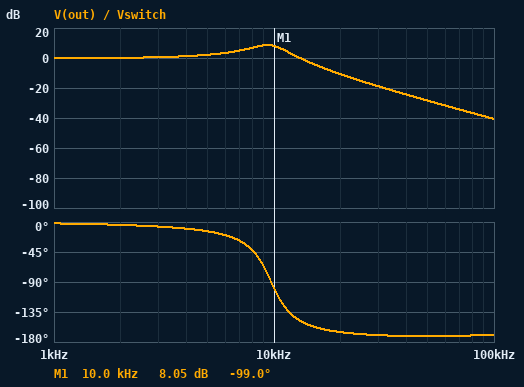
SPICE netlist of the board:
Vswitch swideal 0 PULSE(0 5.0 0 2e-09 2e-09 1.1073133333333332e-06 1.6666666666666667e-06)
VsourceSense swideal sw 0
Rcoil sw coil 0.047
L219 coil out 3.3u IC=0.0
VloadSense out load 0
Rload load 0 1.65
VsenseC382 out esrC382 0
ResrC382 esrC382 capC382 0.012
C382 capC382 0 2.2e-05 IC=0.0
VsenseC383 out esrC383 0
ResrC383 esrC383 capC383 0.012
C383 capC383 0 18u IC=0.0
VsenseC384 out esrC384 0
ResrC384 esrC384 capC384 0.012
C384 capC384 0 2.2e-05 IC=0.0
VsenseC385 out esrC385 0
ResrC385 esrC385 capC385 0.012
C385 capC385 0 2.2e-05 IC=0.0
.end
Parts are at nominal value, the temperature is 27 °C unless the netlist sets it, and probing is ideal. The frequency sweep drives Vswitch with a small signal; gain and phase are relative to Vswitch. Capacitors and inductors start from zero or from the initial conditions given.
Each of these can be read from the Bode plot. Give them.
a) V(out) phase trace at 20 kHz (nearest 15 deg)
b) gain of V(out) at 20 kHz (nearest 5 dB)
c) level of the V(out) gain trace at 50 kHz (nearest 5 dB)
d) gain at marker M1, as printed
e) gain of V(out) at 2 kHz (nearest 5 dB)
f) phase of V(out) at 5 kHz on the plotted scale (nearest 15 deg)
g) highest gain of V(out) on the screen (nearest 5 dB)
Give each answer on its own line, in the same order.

-165 deg
-10 dB
-30 dB
8.05 dB
0 dB
-15 deg
10 dB
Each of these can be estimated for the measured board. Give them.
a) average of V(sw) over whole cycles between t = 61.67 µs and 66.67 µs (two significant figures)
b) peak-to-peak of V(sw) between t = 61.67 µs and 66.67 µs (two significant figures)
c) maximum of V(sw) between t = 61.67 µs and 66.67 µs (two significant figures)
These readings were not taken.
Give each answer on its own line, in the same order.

3.3 V
5.0 V
5.0 V
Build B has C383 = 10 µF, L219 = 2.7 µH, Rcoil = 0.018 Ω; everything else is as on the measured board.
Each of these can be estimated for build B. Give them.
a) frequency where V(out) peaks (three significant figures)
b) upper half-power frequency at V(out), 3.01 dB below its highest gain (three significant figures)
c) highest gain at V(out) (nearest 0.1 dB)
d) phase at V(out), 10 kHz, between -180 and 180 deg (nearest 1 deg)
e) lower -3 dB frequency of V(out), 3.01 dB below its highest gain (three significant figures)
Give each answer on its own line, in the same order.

11.0 kHz
12.2 kHz
12.9 dB
-45 deg
9.67 kHz
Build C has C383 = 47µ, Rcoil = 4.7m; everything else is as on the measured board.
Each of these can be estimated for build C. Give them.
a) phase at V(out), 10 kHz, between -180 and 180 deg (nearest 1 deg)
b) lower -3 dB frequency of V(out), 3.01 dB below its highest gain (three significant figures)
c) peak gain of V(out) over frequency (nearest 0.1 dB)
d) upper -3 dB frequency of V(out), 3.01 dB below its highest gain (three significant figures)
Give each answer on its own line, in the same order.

-157 deg
7.55 kHz
16.4 dB
8.80 kHz
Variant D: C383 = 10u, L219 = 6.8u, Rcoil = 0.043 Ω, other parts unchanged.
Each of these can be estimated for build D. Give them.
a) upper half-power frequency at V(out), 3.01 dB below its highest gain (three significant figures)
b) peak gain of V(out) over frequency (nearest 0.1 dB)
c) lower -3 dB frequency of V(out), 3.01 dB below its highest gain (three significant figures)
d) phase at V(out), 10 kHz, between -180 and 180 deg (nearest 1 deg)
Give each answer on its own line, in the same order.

7.99 kHz
9.5 dB
5.57 kHz
-154 deg
